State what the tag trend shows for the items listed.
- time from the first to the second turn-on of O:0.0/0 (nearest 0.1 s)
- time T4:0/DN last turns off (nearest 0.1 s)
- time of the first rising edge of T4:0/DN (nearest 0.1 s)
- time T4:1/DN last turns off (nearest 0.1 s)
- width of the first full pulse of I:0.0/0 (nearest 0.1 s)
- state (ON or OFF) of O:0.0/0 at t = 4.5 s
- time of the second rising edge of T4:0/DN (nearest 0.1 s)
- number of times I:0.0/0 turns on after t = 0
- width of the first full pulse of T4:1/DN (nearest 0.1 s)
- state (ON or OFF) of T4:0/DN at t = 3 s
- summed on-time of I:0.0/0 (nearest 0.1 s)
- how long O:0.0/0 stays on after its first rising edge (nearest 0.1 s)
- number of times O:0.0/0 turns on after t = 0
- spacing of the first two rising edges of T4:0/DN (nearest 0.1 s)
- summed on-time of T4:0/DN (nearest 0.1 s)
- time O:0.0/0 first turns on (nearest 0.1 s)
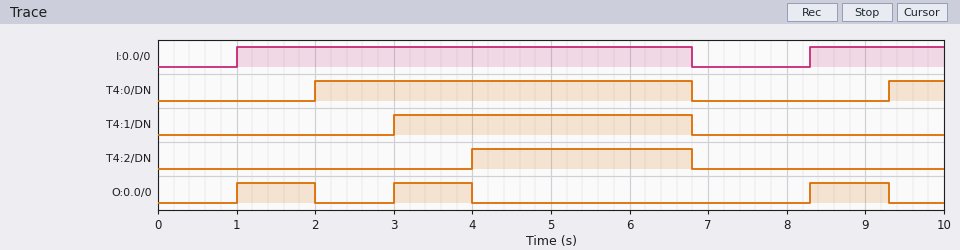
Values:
2.0 s
6.8 s
2.0 s
6.8 s
5.8 s
OFF
9.3 s
2
3.8 s
ON
7.5 s
1.0 s
3
7.3 s
5.5 s
1.0 s
